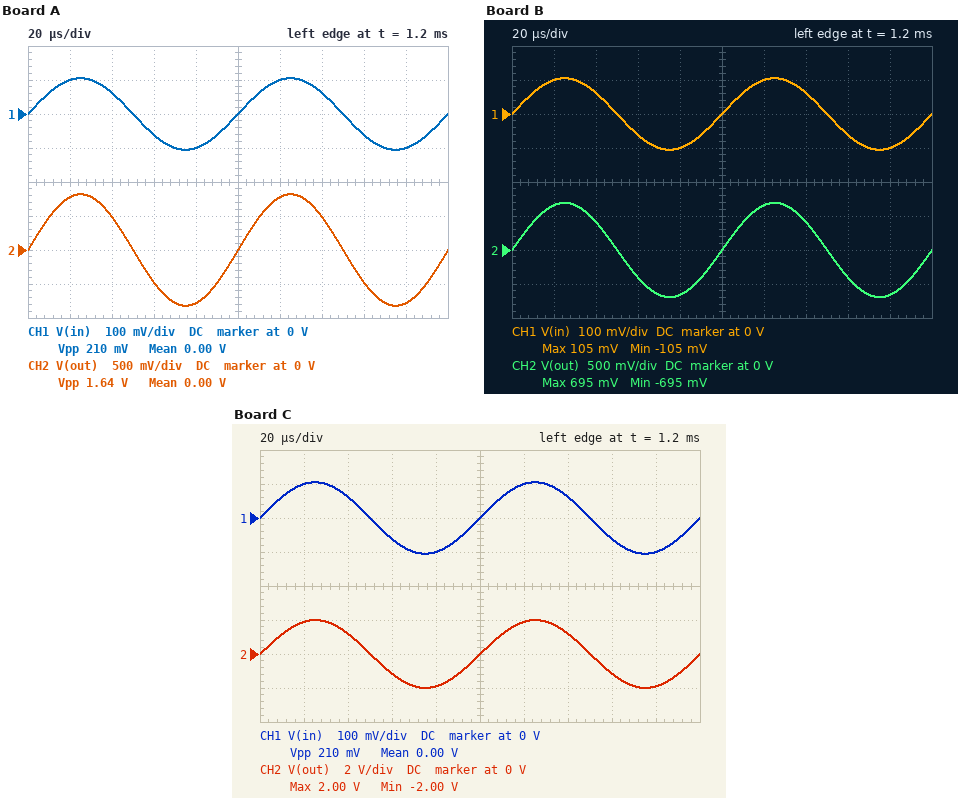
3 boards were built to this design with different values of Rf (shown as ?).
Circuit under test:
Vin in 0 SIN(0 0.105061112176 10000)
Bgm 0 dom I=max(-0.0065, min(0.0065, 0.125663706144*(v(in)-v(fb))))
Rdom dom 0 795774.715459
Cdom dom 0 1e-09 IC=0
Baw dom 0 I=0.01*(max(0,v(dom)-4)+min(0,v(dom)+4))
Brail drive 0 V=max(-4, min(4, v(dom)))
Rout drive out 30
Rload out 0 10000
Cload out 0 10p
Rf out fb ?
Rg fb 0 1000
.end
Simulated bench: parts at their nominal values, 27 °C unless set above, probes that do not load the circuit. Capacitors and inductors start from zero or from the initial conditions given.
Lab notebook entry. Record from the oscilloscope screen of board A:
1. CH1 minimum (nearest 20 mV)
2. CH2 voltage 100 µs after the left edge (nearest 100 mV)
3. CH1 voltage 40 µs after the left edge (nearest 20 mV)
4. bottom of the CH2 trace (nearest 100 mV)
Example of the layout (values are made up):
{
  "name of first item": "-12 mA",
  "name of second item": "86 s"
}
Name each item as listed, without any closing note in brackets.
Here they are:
{
  "CH1 minimum": "-100 mV",
  "CH2 voltage 100 µs after the left edge": "0 V",
  "CH1 voltage 40 µs after the left edge": "60 mV",
  "bottom of the CH2 trace": "-800 mV"
}
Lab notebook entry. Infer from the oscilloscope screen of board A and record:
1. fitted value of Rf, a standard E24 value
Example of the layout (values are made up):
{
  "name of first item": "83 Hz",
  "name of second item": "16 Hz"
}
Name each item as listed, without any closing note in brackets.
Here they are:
{
  "fitted value of Rf, a standard E24 value": "6.8 kΩ"
}
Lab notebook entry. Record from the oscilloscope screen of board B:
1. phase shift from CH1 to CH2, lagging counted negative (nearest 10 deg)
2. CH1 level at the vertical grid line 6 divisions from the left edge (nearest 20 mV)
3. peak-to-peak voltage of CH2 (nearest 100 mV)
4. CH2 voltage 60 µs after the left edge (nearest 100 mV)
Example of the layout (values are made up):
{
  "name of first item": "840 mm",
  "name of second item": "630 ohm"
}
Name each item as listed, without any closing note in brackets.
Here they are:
{
  "phase shift from CH1 to CH2, lagging counted negative": "0 deg",
  "CH1 level at the vertical grid line 6 divisions from the left edge": "100 mV",
  "peak-to-peak voltage of CH2": "1.4 V",
  "CH2 voltage 60 µs after the left edge": "-400 mV"
}
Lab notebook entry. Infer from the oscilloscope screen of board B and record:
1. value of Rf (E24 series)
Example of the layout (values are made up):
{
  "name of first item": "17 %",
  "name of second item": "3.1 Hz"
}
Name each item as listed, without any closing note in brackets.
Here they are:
{
  "value of Rf": "5.6 kΩ"
}
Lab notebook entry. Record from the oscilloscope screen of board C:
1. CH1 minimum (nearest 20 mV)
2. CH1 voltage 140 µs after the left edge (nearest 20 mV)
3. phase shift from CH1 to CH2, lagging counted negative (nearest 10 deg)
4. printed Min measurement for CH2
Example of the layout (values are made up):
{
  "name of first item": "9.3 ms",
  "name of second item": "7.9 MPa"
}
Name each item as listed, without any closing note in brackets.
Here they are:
{
  "CH1 minimum": "-100 mV",
  "CH1 voltage 140 µs after the left edge": "60 mV",
  "phase shift from CH1 to CH2, lagging counted negative": "0 deg",
  "printed Min measurement for CH2": "-2.00 V"
}
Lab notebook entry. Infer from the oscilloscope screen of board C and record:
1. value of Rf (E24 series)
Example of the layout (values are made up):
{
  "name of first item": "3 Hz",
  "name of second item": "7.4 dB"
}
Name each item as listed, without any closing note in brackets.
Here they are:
{
  "value of Rf": "18 kΩ"
}
